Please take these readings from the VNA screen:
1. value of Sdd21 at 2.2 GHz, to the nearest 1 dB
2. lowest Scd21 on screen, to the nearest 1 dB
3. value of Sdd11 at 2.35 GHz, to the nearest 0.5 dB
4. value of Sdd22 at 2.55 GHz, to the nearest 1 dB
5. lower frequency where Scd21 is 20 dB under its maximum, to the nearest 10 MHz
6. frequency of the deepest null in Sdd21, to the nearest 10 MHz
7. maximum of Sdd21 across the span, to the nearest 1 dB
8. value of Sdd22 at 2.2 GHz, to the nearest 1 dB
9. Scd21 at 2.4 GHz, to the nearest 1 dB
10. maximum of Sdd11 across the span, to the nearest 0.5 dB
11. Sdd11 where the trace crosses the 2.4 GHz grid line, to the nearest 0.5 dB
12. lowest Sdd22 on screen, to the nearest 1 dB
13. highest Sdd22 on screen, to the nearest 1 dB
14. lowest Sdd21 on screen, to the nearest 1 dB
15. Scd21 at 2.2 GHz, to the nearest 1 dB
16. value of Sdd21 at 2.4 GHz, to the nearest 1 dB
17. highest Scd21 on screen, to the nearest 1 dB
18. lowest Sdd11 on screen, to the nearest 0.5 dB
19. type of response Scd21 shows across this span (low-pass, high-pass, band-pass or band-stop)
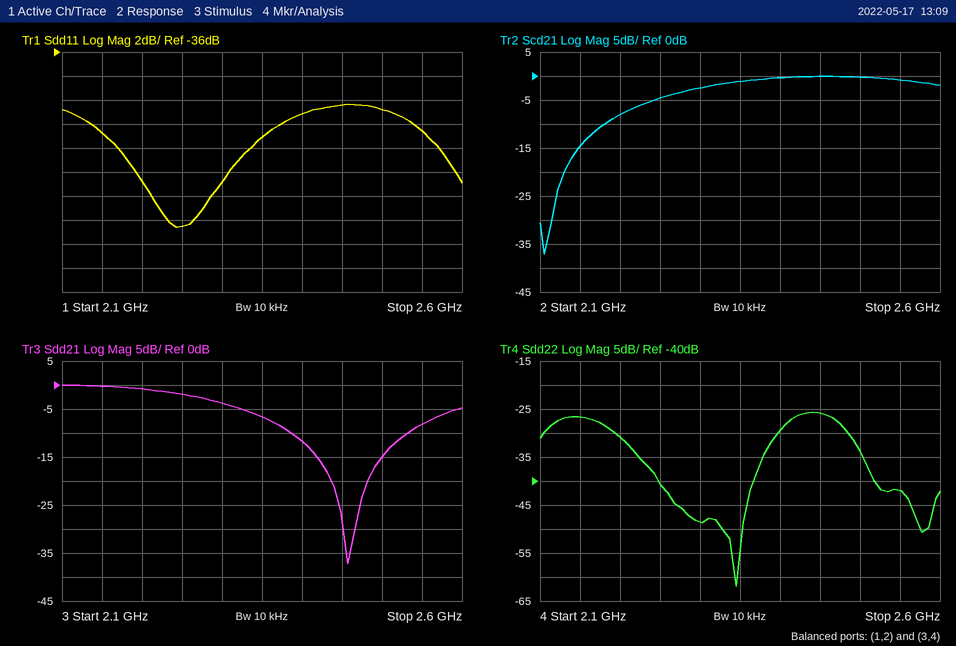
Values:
-1 dB
-37 dB
-43.0 dB
-42 dB
2.13 GHz
2.46 GHz
0 dB
-31 dB
0 dB
-40.5 dB
-41.0 dB
-62 dB
-26 dB
-37 dB
-8 dB
-12 dB
0 dB
-50.5 dB
high-pass
